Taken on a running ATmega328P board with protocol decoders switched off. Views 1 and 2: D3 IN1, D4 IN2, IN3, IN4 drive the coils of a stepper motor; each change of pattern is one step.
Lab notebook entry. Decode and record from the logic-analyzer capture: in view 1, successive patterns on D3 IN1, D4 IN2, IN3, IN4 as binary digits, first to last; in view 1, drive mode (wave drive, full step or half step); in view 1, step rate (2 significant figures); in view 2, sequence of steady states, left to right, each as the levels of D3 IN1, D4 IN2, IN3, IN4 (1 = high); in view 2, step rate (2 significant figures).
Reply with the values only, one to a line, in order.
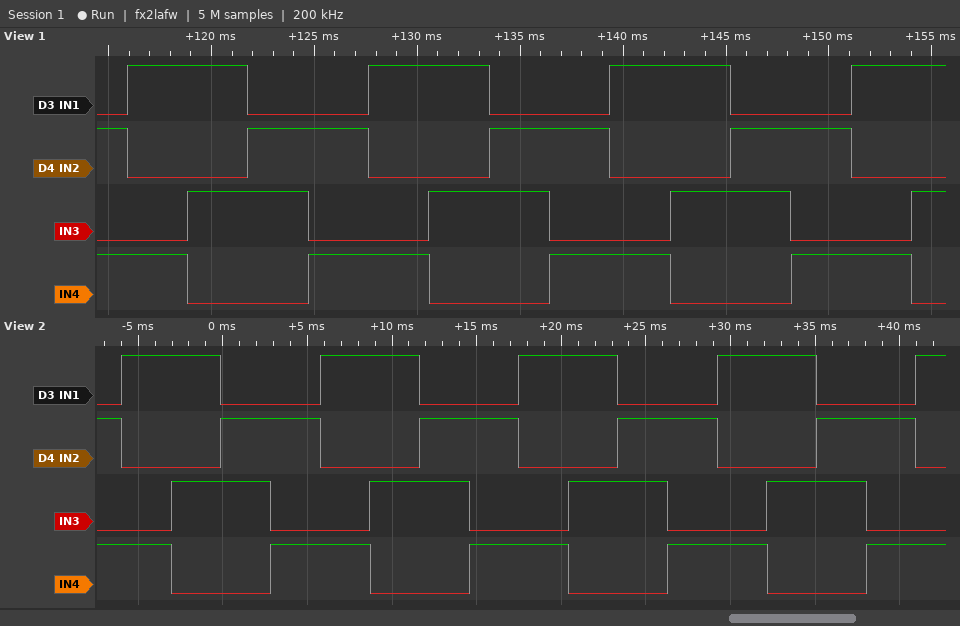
0101 1001 1010 0110 0101 1001 1010 0110 0101 1001 1010 0110 0101 1001 1010
full step
340 steps/s
0101 1001 1010 0110 0101 1001 1010 0110 0101 1001 1010 0110 0101 1001 1010 0110 0101 1001
340 steps/s
